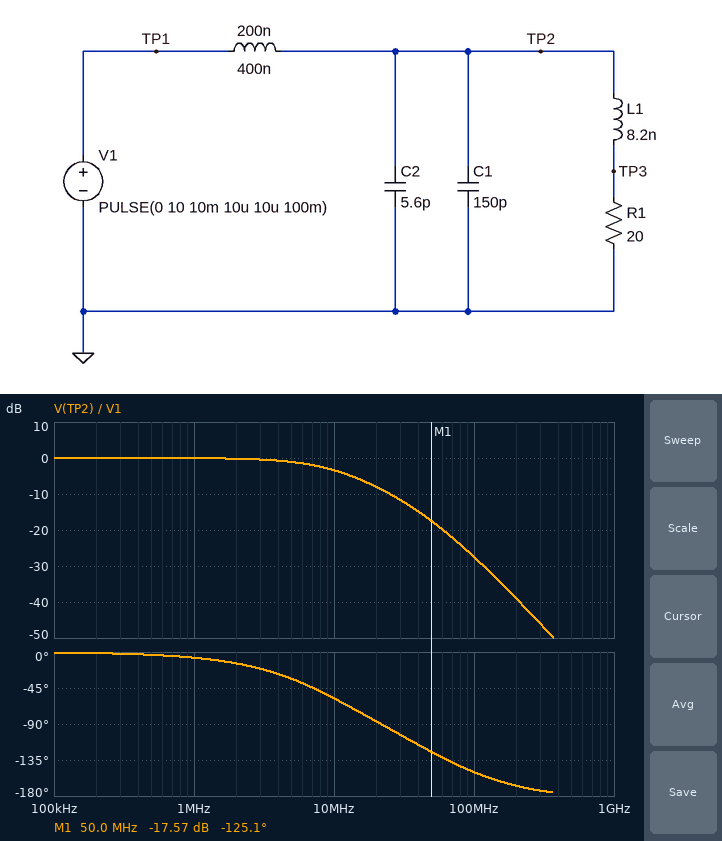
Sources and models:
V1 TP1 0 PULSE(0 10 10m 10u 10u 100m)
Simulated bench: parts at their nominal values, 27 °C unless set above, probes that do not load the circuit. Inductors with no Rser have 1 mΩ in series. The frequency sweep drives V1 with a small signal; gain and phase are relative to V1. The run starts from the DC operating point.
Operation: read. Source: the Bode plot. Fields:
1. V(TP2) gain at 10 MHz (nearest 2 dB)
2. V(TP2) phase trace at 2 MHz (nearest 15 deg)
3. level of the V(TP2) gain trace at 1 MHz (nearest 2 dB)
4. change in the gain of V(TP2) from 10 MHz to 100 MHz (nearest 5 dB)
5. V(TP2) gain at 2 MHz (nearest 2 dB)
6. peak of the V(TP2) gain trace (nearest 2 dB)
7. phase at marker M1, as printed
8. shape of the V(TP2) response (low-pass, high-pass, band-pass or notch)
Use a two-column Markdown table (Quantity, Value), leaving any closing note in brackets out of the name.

| Quantity | Value |
|---|---|
| V(TP2) gain at 10 MHz | -4 dB |
| V(TP2) phase trace at 2 MHz | -15 deg |
| level of the V(TP2) gain trace at 1 MHz | 0 dB |
| change in the gain of V(TP2) from 10 MHz to 100 MHz | -25 dB |
| V(TP2) gain at 2 MHz | 0 dB |
| peak of the V(TP2) gain trace | 0 dB |
| phase at marker M1, as printed | -125.1 deg |
| shape of the V(TP2) response | low-pass |
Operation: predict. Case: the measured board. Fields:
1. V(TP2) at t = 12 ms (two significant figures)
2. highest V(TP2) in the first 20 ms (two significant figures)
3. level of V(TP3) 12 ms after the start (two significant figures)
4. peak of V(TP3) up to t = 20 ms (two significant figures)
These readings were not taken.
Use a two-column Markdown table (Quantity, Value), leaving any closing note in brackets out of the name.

| Quantity | Value |
|---|---|
| V(TP2) at t = 12 ms | 10 V |
| highest V(TP2) in the first 20 ms | 10 V |
| level of V(TP3) 12 ms after the start | 10 V |
| peak of V(TP3) up to t = 20 ms | 10 V |
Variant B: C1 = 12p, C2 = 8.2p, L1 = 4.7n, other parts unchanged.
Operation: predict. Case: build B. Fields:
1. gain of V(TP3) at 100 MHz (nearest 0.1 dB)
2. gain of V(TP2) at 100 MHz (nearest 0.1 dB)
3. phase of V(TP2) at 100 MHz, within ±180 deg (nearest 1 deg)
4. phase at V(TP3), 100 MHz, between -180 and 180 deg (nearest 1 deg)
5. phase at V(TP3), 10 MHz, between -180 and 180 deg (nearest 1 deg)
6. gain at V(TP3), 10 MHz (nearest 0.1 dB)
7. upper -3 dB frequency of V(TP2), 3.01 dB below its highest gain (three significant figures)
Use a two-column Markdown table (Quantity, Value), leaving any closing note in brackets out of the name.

| Quantity | Value |
|---|---|
| gain of V(TP3) at 100 MHz | -21.9 dB |
| gain of V(TP2) at 100 MHz | -21.8 dB |
| phase of V(TP2) at 100 MHz, within ±180 deg | -92 deg |
| phase at V(TP3), 100 MHz, between -180 and 180 deg | -100 deg |
| phase at V(TP3), 10 MHz, between -180 and 180 deg | -53 deg |
| gain at V(TP3), 10 MHz | -4.1 dB |
| upper -3 dB frequency of V(TP2), 3.01 dB below its highest gain | 8.03 MHz |
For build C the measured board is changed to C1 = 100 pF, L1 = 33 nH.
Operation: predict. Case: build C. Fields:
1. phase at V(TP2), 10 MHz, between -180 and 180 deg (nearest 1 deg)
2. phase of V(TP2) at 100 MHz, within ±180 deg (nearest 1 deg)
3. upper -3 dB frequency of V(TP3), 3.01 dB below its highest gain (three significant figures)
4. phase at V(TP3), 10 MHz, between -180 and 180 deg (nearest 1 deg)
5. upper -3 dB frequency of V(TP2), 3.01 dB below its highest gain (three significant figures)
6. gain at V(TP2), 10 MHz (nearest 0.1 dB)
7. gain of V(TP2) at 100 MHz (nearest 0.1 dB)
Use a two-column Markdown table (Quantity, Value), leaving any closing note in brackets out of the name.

| Quantity | Value |
|---|---|
| phase at V(TP2), 10 MHz, between -180 and 180 deg | -52 deg |
| phase of V(TP2) at 100 MHz, within ±180 deg | -147 deg |
| upper -3 dB frequency of V(TP3), 3.01 dB below its highest gain | 8.15 MHz |
| phase at V(TP3), 10 MHz, between -180 and 180 deg | -58 deg |
| upper -3 dB frequency of V(TP2), 3.01 dB below its highest gain | 8.21 MHz |
| gain at V(TP2), 10 MHz | -3.9 dB |
| gain of V(TP2) at 100 MHz | -21.0 dB |
